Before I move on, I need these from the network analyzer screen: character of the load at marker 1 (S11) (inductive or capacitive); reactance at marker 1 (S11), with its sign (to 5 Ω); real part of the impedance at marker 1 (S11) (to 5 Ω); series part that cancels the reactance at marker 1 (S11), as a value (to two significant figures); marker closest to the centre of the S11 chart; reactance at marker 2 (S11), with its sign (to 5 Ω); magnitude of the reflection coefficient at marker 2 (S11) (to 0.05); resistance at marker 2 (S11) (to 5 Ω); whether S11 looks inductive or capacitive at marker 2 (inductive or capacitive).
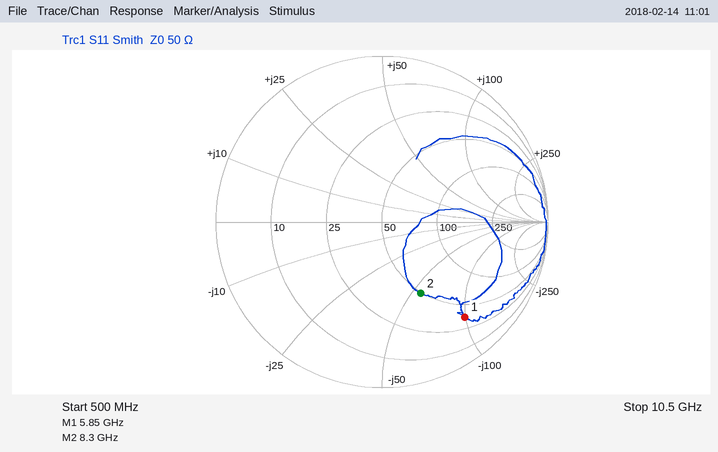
capacitive
-100 Ω
35 Ω
2.7 nH
marker 2
-55 Ω
0.50
50 Ω
capacitive
